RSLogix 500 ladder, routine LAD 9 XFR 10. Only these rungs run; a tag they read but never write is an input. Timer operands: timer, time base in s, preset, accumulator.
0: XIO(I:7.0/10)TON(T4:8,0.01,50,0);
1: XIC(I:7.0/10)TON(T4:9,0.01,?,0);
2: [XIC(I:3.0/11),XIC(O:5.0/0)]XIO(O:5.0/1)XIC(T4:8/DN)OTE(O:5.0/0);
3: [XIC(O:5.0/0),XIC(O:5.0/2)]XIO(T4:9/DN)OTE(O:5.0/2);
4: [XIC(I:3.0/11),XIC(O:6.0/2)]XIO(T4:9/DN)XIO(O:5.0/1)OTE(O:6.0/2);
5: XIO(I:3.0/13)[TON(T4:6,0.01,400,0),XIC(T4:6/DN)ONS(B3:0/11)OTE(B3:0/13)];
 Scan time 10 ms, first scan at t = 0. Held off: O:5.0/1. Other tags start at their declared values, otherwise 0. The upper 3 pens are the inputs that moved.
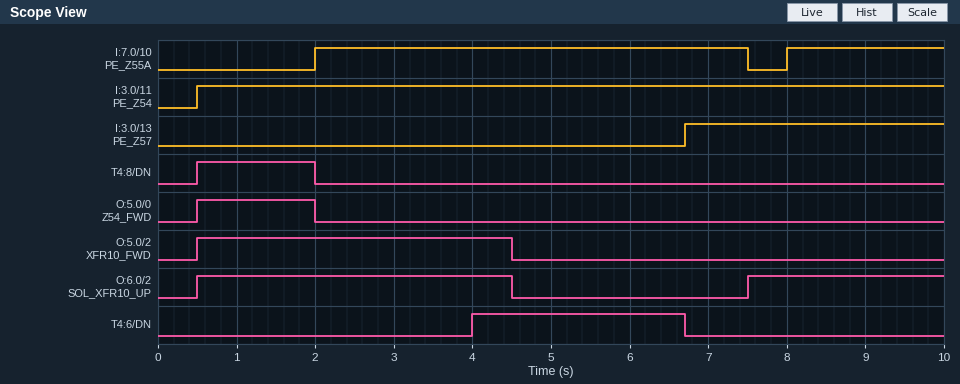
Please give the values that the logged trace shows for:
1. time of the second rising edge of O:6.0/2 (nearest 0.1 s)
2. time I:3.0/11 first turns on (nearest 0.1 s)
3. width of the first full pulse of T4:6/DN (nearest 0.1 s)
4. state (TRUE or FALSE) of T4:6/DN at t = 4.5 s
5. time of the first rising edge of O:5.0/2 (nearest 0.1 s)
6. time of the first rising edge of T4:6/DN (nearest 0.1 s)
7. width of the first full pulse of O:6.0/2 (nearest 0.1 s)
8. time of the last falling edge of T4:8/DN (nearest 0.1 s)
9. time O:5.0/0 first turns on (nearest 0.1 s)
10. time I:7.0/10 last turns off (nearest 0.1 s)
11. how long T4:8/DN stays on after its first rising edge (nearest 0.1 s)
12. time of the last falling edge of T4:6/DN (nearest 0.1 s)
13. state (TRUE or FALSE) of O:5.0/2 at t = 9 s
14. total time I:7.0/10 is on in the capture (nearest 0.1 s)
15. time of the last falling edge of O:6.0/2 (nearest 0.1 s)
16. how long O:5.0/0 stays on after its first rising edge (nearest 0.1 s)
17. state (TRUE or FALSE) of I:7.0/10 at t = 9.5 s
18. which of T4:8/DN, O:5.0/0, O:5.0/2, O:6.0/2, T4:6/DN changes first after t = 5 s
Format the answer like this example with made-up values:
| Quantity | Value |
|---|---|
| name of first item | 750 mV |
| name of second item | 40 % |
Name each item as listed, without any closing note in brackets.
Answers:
| Quantity | Value |
|---|---|
| time of the second rising edge of O:6.0/2 | 7.5 s |
| time I:3.0/11 first turns on | 0.5 s |
| width of the first full pulse of T4:6/DN | 2.7 s |
| state (TRUE or FALSE) of T4:6/DN at t = 4.5 s | TRUE |
| time of the first rising edge of O:5.0/2 | 0.5 s |
| time of the first rising edge of T4:6/DN | 4.0 s |
| width of the first full pulse of O:6.0/2 | 4.0 s |
| time of the last falling edge of T4:8/DN | 2.0 s |
| time O:5.0/0 first turns on | 0.5 s |
| time I:7.0/10 last turns off | 7.5 s |
| how long T4:8/DN stays on after its first rising edge | 1.5 s |
| time of the last falling edge of T4:6/DN | 6.7 s |
| state (TRUE or FALSE) of O:5.0/2 at t = 9 s | FALSE |
| total time I:7.0/10 is on in the capture | 7.5 s |
| time of the last falling edge of O:6.0/2 | 4.5 s |
| how long O:5.0/0 stays on after its first rising edge | 1.5 s |
| state (TRUE or FALSE) of I:7.0/10 at t = 9.5 s | TRUE |
| which of T4:8/DN, O:5.0/0, O:5.0/2, O:6.0/2, T4:6/DN changes first after t = 5 s | T4:6/DN |
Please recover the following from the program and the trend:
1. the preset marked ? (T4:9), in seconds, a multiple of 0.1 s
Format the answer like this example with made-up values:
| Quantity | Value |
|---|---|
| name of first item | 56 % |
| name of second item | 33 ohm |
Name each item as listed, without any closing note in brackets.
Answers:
| Quantity | Value |
|---|---|
| the preset marked ? (T4:9), in seconds, a multiple of 0.1 s | 2.5 s |
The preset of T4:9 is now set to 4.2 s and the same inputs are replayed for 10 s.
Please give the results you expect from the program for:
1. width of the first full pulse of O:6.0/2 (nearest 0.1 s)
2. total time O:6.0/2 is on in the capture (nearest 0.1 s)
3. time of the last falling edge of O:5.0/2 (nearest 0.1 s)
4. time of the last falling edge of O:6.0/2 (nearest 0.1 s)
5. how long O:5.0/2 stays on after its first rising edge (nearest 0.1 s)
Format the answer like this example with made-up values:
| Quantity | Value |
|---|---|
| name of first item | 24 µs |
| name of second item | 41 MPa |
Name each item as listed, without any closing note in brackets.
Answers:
| Quantity | Value |
|---|---|
| width of the first full pulse of O:6.0/2 | 5.7 s |
| total time O:6.0/2 is on in the capture | 8.2 s |
| time of the last falling edge of O:5.0/2 | 6.2 s |
| time of the last falling edge of O:6.0/2 | 6.2 s |
| how long O:5.0/2 stays on after its first rising edge | 5.7 s |
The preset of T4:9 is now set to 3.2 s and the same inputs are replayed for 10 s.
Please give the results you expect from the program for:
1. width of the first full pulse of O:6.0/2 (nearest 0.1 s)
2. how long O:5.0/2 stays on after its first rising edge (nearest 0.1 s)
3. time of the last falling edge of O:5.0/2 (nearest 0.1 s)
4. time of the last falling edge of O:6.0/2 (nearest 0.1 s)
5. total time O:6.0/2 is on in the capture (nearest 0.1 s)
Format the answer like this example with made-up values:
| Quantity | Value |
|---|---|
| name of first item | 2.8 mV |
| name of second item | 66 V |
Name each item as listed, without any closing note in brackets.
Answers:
| Quantity | Value |
|---|---|
| width of the first full pulse of O:6.0/2 | 4.7 s |
| how long O:5.0/2 stays on after its first rising edge | 4.7 s |
| time of the last falling edge of O:5.0/2 | 5.2 s |
| time of the last falling edge of O:6.0/2 | 5.2 s |
| total time O:6.0/2 is on in the capture | 7.2 s |
